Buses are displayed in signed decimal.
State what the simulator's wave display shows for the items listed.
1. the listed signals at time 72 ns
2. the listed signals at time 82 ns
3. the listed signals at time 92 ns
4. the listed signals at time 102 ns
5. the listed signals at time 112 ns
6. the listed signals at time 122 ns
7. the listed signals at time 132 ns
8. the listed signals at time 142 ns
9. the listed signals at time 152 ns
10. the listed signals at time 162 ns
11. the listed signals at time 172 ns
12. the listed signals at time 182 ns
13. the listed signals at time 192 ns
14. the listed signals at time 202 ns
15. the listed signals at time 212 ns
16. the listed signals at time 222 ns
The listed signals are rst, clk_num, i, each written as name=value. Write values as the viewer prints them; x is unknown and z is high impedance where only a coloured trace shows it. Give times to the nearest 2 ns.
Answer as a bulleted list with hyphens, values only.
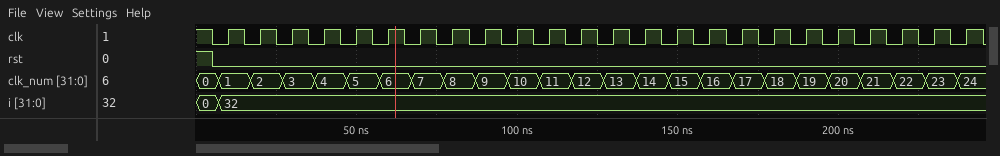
- rst=0, clk_num=7, i=32
- rst=0, clk_num=8, i=32
- rst=0, clk_num=9, i=32
- rst=0, clk_num=10, i=32
- rst=0, clk_num=11, i=32
- rst=0, clk_num=12, i=32
- rst=0, clk_num=13, i=32
- rst=0, clk_num=14, i=32
- rst=0, clk_num=15, i=32
- rst=0, clk_num=16, i=32
- rst=0, clk_num=17, i=32
- rst=0, clk_num=18, i=32
- rst=0, clk_num=19, i=32
- rst=0, clk_num=20, i=32
- rst=0, clk_num=21, i=32
- rst=0, clk_num=22, i=32
